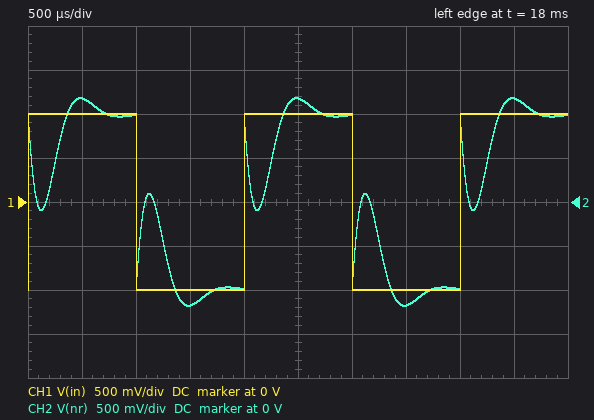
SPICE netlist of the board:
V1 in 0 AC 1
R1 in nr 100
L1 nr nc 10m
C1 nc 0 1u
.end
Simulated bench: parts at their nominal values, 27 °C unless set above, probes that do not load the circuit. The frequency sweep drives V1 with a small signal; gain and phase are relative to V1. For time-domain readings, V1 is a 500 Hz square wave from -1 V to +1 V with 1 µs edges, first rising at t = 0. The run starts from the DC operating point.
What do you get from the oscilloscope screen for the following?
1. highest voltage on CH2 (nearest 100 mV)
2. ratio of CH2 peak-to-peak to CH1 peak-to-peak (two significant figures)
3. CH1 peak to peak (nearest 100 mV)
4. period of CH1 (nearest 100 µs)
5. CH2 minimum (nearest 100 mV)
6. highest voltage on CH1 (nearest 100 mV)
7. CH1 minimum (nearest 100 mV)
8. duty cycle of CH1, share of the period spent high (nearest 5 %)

1.2 V
1.2
2.0 V
2.0 ms
-1.2 V
1.0 V
-1.0 V
50 %
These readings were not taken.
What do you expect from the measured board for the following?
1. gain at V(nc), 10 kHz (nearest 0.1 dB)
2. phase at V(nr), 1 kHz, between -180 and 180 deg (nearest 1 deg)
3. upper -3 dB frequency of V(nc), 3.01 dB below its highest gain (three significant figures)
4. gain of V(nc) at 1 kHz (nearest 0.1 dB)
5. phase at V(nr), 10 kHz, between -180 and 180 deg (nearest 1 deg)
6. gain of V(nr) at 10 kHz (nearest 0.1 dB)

-31.8 dB
-46 deg
1.86 kHz
1.2 dB
9 deg
-0.1 dB
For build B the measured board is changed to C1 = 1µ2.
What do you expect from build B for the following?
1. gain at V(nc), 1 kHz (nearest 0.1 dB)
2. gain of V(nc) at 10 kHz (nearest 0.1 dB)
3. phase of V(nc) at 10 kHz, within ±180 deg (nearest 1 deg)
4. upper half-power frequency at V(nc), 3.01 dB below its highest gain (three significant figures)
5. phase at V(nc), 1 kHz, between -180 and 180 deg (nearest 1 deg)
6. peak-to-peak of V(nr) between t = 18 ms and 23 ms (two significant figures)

0.7 dB
-33.4 dB
-171 deg
1.67 kHz
-55 deg
2.3 V
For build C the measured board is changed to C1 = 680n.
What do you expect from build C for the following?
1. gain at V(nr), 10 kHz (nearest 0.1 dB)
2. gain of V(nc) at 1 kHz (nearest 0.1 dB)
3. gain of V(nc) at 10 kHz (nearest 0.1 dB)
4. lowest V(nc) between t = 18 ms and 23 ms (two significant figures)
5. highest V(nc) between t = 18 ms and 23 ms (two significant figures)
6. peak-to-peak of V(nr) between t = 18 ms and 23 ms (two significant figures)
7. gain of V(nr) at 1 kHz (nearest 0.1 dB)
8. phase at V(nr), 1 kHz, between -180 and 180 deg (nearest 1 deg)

-0.1 dB
1.4 dB
-28.4 dB
-1.5 V
1.5 V
2.5 V
-1.3 dB
-30 deg
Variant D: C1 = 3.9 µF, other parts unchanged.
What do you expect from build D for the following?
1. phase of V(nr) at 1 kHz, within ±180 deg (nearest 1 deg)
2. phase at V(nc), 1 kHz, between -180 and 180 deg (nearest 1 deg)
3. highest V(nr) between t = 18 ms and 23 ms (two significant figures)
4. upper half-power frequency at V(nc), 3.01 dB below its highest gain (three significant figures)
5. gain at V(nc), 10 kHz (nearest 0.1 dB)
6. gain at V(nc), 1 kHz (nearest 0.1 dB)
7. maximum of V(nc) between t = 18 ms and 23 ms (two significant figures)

78 deg
-102 deg
1.1 V
528 Hz
-43.8 dB
-8.0 dB
930 mV
